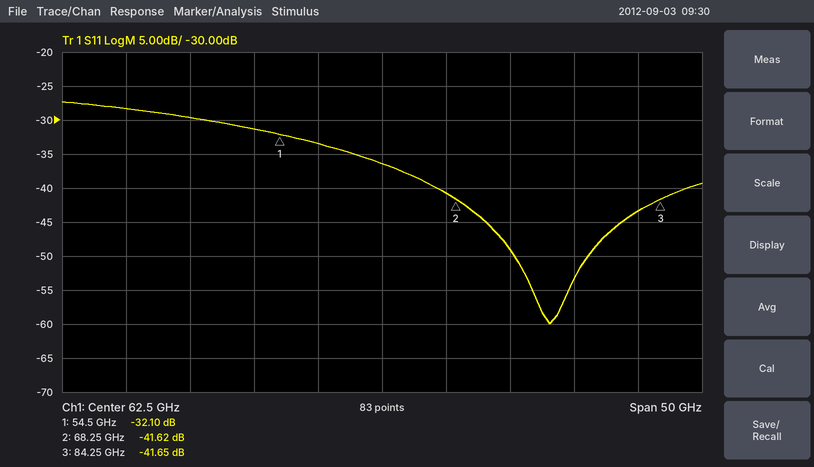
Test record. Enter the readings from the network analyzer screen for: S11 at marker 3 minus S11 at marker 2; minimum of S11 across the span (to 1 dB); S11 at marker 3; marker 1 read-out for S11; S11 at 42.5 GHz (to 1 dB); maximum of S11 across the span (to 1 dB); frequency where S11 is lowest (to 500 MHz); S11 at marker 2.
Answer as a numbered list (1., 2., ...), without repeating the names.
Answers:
1. -0.03 dB
2. -60 dB
3. -41.65 dB
4. -32.10 dB
5. -28 dB
6. -27 dB
7. 75.5 GHz
8. -41.62 dB
